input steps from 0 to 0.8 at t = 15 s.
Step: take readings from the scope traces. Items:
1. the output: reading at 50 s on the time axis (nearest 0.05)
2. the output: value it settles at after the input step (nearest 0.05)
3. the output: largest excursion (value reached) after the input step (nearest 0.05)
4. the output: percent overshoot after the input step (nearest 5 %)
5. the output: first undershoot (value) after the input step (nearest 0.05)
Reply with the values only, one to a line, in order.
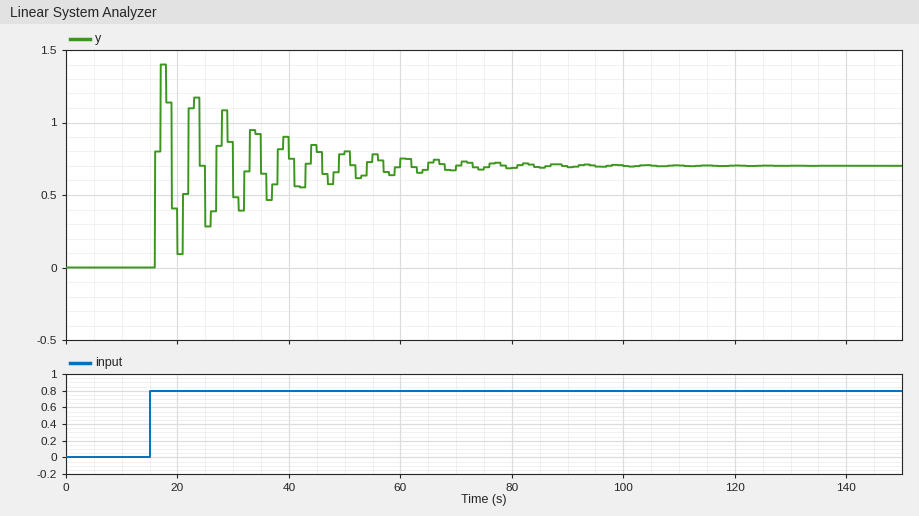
0.80
0.70
1.40
100 %
0.10
